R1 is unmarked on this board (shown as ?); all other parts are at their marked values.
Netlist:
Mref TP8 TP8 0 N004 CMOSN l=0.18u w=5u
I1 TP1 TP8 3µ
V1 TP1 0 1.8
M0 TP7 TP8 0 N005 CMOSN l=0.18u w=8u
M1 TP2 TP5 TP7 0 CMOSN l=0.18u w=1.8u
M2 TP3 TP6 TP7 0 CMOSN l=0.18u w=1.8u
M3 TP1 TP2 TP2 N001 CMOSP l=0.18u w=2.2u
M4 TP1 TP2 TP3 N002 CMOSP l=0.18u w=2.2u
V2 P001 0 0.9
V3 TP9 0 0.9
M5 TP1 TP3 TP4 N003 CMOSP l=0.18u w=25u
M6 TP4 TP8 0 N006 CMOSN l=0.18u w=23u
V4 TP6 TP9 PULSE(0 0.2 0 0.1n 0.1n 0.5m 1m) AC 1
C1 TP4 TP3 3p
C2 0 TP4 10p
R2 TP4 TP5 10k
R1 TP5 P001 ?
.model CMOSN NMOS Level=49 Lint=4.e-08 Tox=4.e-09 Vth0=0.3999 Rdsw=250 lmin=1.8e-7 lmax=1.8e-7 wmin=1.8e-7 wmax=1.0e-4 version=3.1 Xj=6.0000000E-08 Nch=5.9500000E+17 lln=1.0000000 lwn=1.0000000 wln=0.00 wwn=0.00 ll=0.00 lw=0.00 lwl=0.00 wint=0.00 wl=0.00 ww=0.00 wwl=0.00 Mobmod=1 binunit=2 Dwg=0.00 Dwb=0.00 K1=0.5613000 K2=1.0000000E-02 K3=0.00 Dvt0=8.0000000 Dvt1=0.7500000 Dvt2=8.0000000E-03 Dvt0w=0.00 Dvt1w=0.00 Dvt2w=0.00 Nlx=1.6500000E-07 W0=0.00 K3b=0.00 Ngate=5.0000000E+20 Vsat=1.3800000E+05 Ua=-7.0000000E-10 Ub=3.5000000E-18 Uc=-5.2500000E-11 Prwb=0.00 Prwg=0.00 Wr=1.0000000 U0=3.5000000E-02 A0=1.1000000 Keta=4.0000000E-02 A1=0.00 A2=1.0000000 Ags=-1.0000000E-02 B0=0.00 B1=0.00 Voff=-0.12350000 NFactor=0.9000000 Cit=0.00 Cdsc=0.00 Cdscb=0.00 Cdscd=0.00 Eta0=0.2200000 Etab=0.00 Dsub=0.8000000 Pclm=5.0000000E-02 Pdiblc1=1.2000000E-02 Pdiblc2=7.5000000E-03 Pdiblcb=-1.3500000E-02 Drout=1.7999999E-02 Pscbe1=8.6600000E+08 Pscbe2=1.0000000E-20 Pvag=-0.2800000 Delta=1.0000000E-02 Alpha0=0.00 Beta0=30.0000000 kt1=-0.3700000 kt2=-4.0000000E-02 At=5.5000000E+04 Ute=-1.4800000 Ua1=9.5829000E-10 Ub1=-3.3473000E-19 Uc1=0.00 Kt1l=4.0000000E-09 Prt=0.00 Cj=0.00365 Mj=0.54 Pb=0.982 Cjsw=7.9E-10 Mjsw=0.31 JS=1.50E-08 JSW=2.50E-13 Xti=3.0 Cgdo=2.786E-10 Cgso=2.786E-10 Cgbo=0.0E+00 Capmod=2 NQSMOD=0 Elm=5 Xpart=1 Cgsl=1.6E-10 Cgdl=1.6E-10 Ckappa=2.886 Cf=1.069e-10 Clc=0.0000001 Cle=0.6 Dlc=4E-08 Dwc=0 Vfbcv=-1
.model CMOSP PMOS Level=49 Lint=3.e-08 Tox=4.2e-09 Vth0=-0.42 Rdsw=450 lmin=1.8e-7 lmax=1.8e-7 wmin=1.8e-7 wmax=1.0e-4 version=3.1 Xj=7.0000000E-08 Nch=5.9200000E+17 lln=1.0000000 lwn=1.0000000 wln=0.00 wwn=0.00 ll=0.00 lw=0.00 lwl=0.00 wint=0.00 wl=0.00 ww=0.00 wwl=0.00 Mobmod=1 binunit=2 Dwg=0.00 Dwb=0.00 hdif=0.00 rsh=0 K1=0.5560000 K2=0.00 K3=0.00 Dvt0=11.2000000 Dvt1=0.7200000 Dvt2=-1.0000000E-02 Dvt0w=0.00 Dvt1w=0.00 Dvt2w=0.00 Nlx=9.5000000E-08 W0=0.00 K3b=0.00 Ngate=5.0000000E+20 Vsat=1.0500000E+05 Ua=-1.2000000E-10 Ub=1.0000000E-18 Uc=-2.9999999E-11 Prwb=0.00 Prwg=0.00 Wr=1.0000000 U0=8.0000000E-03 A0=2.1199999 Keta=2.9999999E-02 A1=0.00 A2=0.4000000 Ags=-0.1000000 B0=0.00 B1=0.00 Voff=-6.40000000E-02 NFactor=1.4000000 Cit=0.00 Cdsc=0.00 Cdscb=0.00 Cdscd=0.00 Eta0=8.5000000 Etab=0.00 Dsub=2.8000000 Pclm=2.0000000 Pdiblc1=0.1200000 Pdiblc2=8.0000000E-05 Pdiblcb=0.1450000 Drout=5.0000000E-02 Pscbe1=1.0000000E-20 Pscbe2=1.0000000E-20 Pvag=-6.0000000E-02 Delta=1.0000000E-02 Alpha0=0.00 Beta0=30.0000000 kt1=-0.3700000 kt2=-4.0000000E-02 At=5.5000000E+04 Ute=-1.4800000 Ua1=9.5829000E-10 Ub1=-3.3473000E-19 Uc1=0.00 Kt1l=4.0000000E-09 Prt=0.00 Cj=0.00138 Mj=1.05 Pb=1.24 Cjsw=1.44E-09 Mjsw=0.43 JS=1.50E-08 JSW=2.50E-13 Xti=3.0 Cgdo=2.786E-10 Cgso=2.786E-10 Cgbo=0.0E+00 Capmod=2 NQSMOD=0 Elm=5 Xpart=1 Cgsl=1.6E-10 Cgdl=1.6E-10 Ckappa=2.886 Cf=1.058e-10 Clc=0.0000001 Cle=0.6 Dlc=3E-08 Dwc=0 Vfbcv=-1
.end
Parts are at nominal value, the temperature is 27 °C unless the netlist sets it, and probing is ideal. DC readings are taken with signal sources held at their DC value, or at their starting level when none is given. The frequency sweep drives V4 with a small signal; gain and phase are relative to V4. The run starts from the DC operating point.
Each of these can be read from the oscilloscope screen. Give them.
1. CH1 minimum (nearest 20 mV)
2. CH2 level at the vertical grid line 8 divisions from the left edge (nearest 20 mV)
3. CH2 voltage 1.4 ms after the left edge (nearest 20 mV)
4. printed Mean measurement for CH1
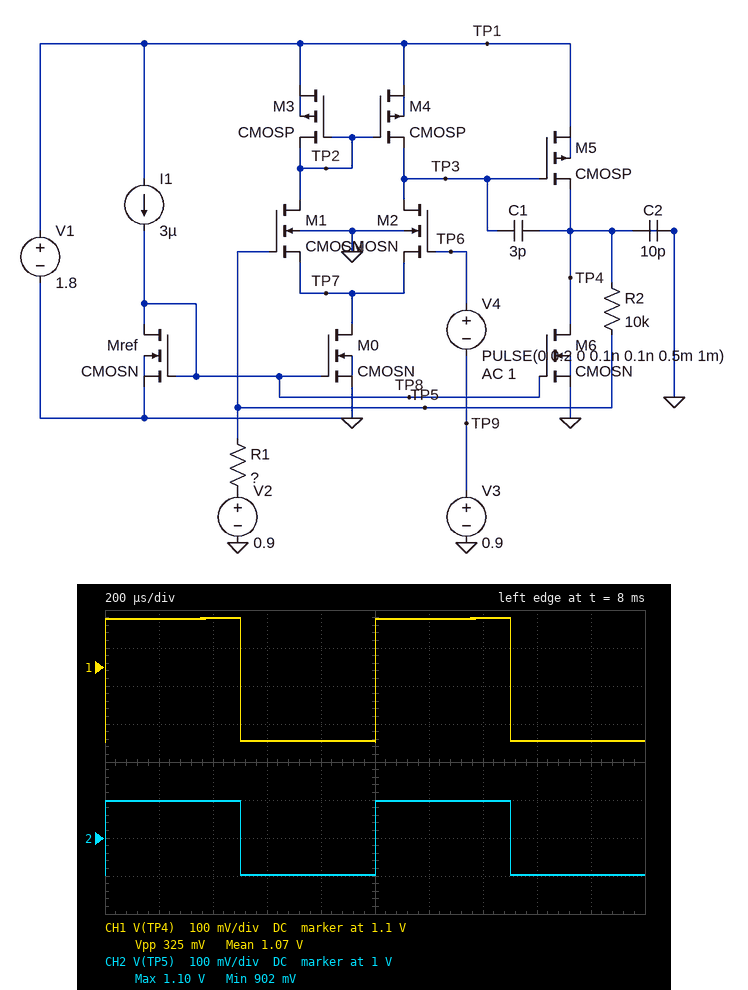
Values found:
900 mV
900 mV
1.10 V
1.07 V
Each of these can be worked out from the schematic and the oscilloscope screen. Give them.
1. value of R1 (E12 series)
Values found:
15 kΩ
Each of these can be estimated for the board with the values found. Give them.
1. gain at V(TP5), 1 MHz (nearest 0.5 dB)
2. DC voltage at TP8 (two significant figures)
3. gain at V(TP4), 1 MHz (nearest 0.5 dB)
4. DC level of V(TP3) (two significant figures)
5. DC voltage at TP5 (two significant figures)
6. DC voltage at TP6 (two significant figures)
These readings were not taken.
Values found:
-1.0 dB
310 mV
3.5 dB
1.5 V
900 mV
900 mV
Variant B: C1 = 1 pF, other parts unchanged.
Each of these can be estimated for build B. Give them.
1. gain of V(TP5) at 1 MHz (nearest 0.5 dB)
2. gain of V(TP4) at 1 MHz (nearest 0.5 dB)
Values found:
-0.5 dB
4.0 dB
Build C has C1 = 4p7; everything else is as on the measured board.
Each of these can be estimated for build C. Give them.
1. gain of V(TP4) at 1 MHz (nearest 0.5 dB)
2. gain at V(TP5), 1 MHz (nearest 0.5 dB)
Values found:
2.5 dB
-2.0 dB
